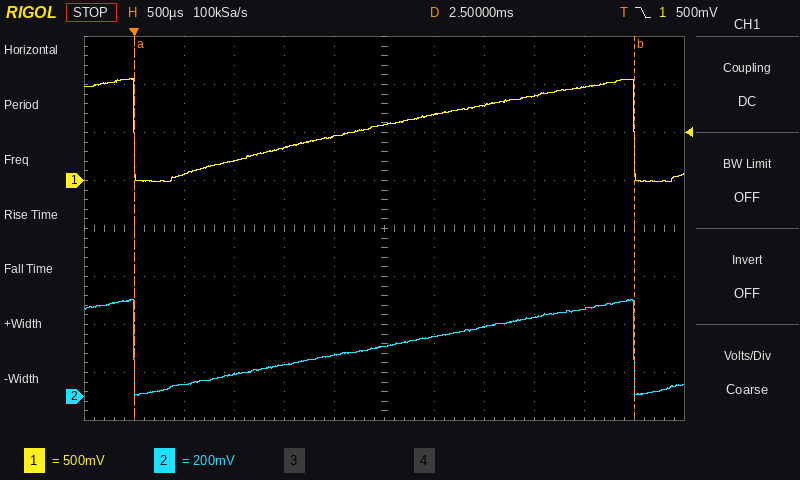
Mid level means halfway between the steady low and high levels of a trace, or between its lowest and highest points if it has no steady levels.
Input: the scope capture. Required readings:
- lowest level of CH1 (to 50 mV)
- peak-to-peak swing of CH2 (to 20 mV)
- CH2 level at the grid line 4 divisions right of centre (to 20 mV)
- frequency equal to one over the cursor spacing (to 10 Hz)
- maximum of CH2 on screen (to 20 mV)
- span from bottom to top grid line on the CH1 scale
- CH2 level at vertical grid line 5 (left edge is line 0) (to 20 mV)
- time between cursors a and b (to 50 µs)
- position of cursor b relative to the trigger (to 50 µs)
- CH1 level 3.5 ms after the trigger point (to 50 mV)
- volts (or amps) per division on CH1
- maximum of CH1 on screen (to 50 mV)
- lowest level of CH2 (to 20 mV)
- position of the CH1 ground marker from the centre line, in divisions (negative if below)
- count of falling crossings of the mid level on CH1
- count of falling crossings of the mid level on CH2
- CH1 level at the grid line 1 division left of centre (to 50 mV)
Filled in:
0 mV
400 mV
360 mV
200 Hz
400 mV
4 V
180 mV
5.00 ms
+5.00 ms
800 mV
500 mV
1.05 V
0 mV
+1.0 div
2
2
450 mV
